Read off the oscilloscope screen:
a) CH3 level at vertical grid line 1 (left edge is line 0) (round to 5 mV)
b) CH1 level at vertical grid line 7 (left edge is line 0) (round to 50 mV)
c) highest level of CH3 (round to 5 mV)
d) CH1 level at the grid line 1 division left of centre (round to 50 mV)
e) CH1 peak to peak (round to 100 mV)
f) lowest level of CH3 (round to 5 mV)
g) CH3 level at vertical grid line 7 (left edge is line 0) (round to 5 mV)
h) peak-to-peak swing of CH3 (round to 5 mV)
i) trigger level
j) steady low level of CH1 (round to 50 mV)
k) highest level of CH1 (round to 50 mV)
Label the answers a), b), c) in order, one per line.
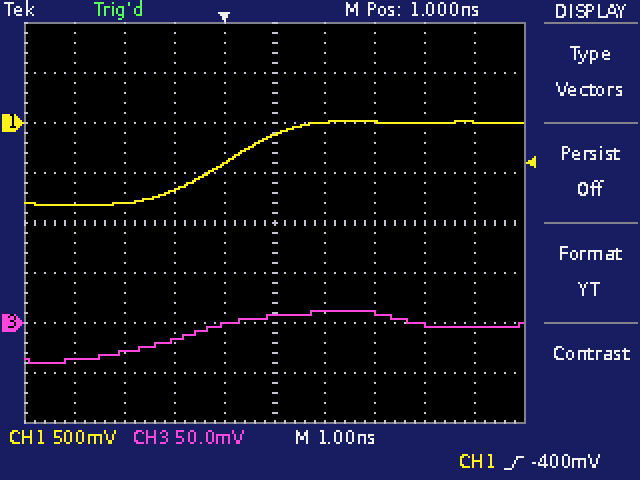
a) -35 mV
b) 0 mV
c) 10 mV
d) -400 mV
e) 800 mV
f) -40 mV
g) 10 mV
h) 50 mV
i) -400 mV
j) -800 mV
k) 0 mV
